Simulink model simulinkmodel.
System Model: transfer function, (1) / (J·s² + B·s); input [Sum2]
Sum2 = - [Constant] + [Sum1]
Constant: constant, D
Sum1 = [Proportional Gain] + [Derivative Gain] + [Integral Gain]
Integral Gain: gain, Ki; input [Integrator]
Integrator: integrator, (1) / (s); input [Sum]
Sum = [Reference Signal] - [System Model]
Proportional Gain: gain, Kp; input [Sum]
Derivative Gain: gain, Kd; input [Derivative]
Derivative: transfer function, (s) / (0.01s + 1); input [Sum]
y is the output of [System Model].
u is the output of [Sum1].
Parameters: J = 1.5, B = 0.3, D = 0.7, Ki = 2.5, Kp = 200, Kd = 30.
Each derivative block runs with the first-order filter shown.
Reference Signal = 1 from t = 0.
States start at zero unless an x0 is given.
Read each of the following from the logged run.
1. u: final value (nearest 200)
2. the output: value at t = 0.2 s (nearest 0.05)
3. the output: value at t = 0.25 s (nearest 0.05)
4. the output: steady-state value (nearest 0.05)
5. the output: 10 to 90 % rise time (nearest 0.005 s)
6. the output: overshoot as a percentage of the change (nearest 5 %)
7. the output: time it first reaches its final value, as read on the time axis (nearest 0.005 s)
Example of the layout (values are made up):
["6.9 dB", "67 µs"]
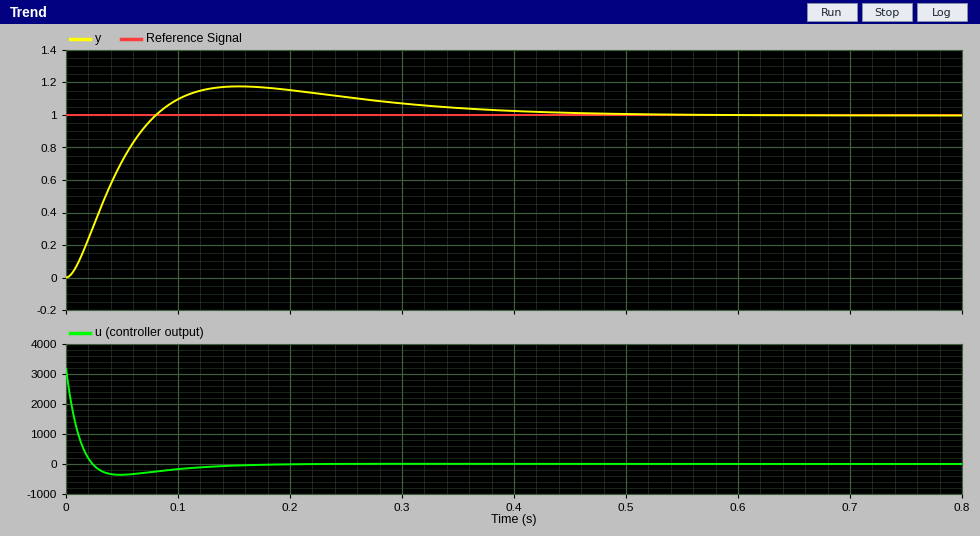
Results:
["0", "1.15", "1.10", "1.00", "0.055 s", "20 %", "0.080 s"]
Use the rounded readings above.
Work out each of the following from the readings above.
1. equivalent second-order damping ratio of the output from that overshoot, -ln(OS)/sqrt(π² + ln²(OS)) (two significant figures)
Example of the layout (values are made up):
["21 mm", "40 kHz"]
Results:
["0.46"]
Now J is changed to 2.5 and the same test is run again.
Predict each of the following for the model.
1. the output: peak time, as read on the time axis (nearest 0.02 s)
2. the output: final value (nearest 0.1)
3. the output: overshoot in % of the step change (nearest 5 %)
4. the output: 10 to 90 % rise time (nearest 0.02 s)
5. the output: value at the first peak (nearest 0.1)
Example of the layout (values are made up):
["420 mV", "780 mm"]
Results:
["0.24 s", "1.0", "25 %", "0.08 s", "1.2"]
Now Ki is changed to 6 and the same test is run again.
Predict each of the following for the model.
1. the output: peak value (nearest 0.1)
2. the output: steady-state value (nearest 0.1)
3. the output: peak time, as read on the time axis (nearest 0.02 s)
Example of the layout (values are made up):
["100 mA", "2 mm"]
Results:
["1.2", "1.0", "0.16 s"]
